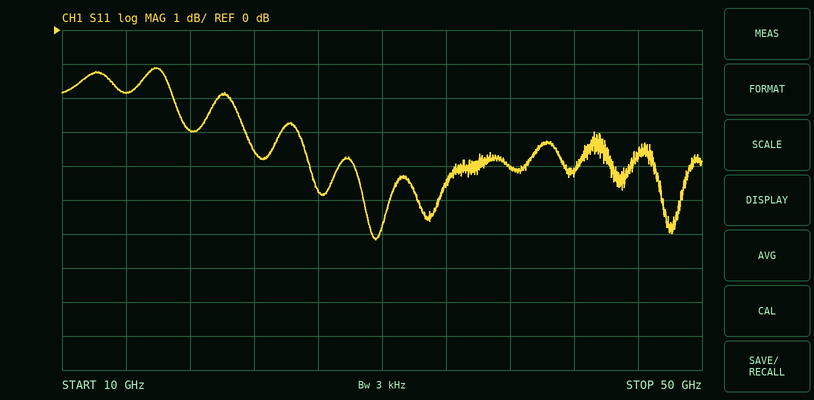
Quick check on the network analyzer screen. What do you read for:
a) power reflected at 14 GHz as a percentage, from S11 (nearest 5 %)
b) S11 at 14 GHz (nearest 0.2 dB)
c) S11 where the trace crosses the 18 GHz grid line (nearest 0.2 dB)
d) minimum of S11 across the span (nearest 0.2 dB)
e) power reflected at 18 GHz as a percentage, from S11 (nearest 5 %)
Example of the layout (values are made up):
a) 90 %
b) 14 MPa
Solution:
a) 65 %
b) -1.8 dB
c) -3.0 dB
d) -6.2 dB
e) 50 %
